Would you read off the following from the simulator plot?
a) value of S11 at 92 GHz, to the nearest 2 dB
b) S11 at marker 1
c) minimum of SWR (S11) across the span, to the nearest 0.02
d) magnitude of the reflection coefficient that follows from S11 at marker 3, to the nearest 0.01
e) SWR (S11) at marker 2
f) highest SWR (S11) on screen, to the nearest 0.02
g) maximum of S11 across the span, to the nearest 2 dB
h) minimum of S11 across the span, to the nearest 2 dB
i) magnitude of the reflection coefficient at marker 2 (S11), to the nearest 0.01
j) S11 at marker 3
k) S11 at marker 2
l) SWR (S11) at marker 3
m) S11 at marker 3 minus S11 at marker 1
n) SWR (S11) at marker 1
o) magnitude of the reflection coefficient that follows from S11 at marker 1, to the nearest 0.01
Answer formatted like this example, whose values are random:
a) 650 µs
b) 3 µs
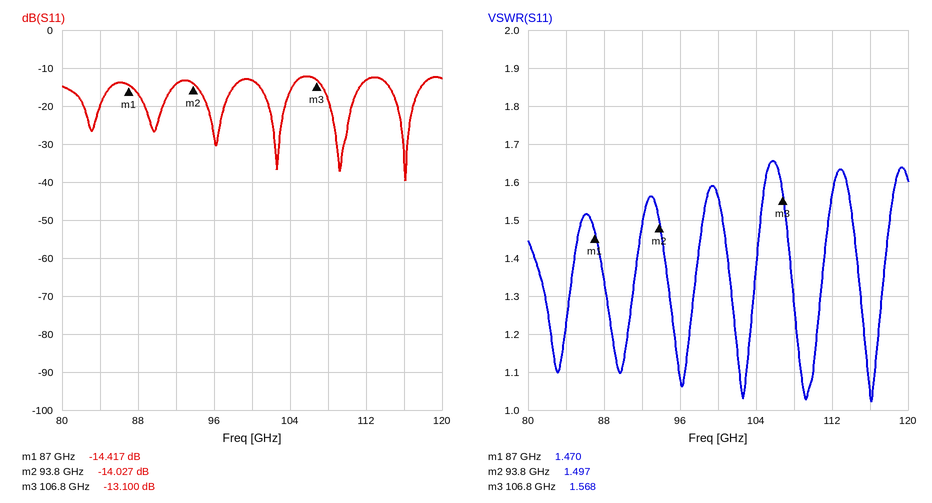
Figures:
a) -14 dB
b) -14.417 dB
c) 1.02
d) 0.22
e) 1.497
f) 1.66
g) -12 dB
h) -40 dB
i) 0.20
j) -13.100 dB
k) -14.027 dB
l) 1.568
m) 1.317 dB
n) 1.470
o) 0.19
